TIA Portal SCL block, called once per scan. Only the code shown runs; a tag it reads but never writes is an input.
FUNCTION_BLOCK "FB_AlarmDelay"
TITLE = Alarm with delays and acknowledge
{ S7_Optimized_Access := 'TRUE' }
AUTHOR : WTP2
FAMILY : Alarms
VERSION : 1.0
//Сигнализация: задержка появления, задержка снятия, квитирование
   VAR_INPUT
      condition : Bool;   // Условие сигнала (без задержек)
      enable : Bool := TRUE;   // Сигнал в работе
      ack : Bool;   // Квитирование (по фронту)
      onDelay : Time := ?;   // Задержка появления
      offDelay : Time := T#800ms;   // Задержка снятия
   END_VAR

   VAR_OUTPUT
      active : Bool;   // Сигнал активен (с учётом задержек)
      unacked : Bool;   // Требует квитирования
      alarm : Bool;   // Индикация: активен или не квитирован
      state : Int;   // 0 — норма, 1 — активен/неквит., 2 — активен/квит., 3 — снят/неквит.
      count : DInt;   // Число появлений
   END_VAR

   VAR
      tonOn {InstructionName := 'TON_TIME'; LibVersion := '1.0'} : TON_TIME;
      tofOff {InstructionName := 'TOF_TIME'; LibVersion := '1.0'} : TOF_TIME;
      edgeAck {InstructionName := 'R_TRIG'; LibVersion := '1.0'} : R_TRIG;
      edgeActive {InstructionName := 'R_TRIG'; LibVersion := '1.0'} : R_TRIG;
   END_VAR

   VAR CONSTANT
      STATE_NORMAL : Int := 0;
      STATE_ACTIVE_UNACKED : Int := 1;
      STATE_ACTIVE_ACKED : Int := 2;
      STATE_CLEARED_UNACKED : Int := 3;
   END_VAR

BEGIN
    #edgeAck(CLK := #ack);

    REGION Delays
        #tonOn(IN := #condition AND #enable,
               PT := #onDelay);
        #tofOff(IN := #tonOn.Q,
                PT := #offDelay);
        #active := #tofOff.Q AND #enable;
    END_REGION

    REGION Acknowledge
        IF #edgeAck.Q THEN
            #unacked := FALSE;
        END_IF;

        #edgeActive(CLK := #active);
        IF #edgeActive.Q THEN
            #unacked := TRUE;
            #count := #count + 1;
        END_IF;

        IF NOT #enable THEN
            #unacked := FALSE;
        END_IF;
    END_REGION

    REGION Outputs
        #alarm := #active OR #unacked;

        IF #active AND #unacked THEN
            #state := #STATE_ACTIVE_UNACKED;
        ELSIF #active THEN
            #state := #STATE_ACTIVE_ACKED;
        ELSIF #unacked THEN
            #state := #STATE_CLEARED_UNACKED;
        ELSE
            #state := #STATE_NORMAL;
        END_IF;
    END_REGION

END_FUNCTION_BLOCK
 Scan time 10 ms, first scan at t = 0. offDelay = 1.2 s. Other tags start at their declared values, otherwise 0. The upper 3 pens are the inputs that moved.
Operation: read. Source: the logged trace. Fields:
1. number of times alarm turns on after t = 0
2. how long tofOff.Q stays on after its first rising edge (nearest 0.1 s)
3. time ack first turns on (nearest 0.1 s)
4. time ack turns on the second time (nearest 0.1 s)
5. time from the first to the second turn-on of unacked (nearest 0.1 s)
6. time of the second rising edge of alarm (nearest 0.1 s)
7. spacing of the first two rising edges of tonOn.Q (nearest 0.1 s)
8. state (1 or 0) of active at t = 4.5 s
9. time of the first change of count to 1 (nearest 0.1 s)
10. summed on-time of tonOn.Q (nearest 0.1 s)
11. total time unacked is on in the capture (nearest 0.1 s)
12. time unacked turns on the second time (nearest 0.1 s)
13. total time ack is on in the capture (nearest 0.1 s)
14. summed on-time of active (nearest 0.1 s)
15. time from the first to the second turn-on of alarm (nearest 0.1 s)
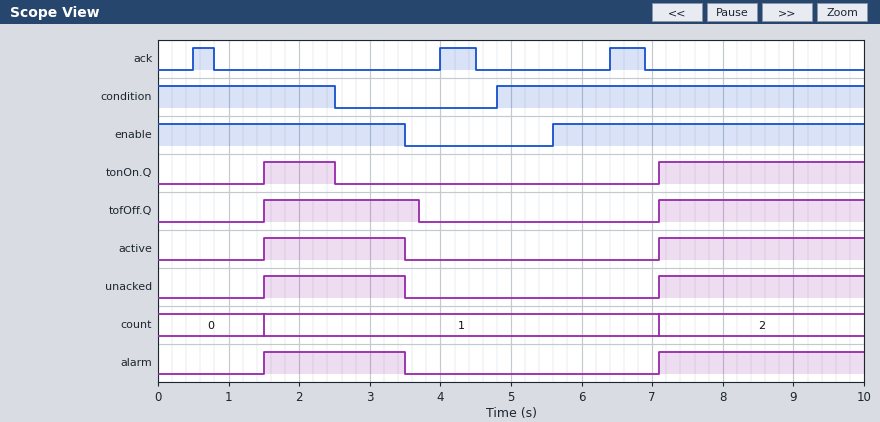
2
2.2 s
0.5 s
4.0 s
5.6 s
7.1 s
5.6 s
0
1.5 s
3.9 s
4.9 s
7.1 s
1.3 s
4.9 s
5.6 s
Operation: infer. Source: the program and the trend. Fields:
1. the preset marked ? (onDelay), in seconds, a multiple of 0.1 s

1.5 s
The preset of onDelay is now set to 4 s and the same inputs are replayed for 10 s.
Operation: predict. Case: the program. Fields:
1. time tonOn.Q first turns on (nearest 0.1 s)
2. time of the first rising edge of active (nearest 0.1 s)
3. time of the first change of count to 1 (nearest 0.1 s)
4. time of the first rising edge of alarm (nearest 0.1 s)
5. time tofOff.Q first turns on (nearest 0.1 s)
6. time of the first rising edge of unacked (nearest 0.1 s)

9.6 s
9.6 s
9.6 s
9.6 s
9.6 s
9.6 s
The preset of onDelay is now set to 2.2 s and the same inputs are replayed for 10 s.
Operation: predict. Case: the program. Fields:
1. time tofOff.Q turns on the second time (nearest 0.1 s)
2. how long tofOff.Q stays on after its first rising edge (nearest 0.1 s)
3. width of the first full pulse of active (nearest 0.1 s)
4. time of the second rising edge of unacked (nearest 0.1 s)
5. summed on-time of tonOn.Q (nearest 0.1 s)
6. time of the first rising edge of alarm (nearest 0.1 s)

7.8 s
1.5 s
1.3 s
7.8 s
2.5 s
2.2 s
